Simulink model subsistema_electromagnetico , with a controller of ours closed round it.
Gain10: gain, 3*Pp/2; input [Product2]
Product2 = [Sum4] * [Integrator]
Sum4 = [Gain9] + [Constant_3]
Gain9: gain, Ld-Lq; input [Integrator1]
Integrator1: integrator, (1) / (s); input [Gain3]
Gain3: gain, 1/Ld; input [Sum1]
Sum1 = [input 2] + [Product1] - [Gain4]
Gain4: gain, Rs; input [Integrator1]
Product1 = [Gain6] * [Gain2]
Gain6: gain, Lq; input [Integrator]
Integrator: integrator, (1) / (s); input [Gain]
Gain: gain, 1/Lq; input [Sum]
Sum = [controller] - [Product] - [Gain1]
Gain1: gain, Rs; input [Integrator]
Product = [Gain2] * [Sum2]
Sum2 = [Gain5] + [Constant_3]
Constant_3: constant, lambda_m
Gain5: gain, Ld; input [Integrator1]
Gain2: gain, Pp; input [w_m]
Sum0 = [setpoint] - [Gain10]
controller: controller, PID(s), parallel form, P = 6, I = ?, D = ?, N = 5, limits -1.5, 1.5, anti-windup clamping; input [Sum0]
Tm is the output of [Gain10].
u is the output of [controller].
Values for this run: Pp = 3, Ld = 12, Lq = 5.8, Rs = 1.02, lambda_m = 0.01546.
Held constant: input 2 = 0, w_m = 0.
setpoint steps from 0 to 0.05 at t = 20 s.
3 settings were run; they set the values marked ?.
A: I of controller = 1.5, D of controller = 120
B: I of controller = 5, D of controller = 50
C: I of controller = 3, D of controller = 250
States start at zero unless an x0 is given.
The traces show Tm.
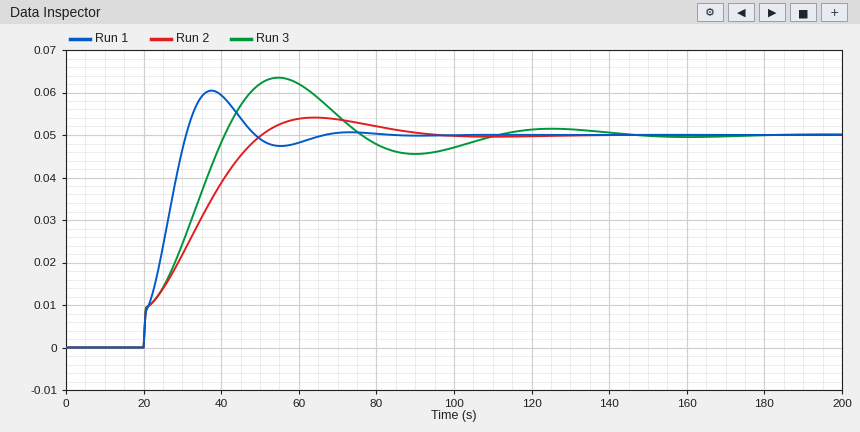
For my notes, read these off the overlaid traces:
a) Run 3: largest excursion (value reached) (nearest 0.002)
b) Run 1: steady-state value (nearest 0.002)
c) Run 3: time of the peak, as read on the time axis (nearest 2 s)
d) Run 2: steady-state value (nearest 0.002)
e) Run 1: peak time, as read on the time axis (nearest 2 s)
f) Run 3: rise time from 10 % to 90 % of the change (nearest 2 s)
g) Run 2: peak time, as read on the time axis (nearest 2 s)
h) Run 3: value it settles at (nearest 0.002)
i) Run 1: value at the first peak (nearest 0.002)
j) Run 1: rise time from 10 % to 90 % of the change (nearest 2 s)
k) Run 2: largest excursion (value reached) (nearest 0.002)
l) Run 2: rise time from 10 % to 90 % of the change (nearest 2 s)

0.064
0.050
54 s
0.050
38 s
18 s
64 s
0.050
0.060
10 s
0.054
24 s
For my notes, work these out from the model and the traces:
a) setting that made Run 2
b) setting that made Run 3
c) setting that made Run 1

A
C
B
